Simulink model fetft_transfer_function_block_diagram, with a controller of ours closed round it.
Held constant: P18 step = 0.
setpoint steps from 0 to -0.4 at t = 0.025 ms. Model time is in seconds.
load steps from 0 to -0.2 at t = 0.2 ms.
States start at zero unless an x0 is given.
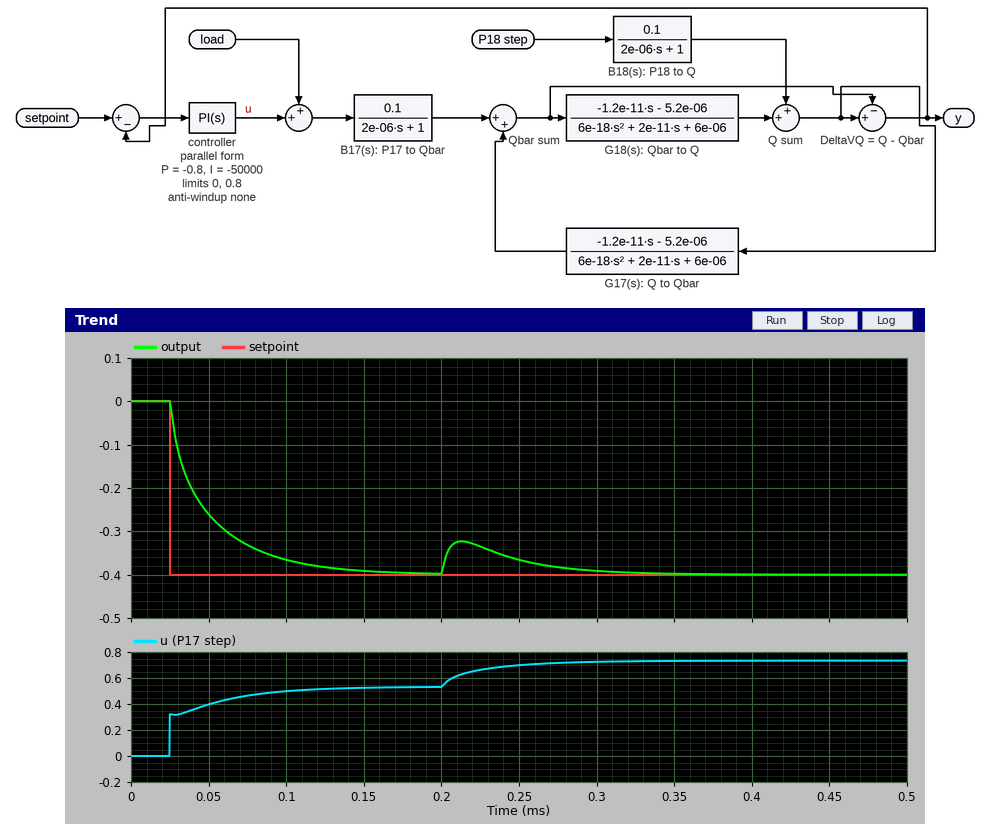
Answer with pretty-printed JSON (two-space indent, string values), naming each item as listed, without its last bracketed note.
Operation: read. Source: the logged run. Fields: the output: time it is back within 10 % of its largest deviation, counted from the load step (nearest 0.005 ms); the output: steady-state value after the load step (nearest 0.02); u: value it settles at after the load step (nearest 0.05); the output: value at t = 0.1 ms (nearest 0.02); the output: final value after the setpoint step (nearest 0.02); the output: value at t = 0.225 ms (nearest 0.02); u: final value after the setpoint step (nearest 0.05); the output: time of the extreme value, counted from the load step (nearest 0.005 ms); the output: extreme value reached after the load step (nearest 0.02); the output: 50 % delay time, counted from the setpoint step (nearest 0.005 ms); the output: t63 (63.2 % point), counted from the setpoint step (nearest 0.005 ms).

{
  "the output: time it is back within 10 % of its largest deviation, counted from the load step": "0.105 ms",
  "the output: steady-state value after the load step": "-0.40",
  "u: value it settles at after the load step": "0.75",
  "the output: value at t = 0.1 ms": "-0.36",
  "the output: final value after the setpoint step": "-0.40",
  "the output: value at t = 0.225 ms": "-0.34",
  "u: final value after the setpoint step": "0.55",
  "the output: time of the extreme value, counted from the load step": "0.015 ms",
  "the output: extreme value reached after the load step": "-0.32",
  "the output: 50 % delay time, counted from the setpoint step": "0.015 ms",
  "the output: t63 (63.2 % point), counted from the setpoint step": "0.025 ms"
}
